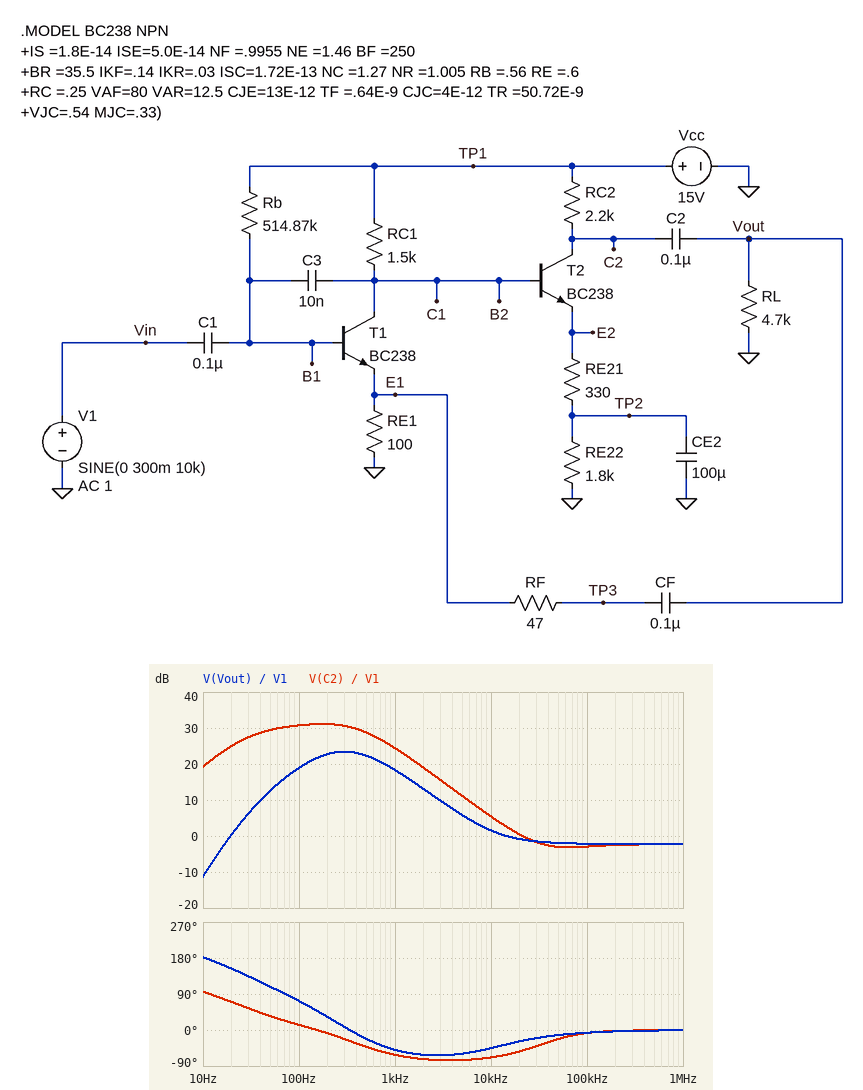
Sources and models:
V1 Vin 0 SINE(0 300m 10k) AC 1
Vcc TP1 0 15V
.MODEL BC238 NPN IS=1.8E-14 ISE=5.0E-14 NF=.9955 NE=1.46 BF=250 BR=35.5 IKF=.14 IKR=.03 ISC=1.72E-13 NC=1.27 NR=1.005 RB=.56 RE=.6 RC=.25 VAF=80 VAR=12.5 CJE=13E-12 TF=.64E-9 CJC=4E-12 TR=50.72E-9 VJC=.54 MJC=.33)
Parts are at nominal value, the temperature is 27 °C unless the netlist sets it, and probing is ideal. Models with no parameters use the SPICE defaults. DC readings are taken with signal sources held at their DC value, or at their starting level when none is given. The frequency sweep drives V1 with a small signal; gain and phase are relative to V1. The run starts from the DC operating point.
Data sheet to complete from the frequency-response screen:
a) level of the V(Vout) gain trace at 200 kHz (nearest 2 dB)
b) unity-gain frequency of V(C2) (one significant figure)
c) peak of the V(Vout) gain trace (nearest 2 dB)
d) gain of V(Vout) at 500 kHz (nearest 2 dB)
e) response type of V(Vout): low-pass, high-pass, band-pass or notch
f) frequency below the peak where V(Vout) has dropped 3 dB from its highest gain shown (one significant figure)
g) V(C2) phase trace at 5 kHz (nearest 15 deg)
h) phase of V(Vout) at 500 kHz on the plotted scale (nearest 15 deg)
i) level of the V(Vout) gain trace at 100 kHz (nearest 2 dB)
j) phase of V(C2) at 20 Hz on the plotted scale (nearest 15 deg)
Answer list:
-2 dB
20 kHz
24 dB
-2 dB
band-pass
100 Hz
-75 deg
0 deg
-2 dB
75 deg
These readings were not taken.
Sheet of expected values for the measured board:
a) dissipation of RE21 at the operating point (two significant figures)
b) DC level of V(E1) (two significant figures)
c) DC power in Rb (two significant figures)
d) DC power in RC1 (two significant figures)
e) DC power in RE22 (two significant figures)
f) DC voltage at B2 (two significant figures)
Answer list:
2.5 mW
570 mV
370 µW
48 mW
14 mW
6.5 V
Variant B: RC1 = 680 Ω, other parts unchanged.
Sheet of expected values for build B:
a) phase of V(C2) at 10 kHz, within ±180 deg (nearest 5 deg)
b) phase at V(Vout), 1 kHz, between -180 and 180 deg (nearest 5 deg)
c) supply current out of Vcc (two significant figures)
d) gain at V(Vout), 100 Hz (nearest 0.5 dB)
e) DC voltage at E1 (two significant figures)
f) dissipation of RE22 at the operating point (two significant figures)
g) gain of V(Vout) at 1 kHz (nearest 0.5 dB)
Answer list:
165 deg
-170 deg
10 mA
-16.0 dB
590 mV
33 mW
-9.5 dB
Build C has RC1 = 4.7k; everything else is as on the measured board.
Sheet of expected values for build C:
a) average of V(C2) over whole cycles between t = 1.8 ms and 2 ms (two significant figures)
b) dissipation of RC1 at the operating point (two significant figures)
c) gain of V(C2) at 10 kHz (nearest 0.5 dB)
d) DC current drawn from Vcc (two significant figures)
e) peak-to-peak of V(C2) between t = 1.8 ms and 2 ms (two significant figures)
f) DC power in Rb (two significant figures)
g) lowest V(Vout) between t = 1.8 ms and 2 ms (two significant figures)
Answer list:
11 V
45 mW
-8.0 dB
3.1 mA
1.2 V
380 µW
-420 mV
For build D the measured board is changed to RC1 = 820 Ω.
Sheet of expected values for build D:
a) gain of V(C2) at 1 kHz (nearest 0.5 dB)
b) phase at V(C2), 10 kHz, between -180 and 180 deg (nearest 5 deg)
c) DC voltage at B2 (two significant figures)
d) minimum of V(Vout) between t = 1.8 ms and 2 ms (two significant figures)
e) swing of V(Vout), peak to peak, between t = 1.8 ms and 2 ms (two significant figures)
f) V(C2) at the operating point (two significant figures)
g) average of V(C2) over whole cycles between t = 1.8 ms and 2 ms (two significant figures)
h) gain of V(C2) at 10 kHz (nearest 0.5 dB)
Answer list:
3.5 dB
165 deg
9.3 V
-140 mV
280 mV
8.6 V
8.8 V
3.0 dB
